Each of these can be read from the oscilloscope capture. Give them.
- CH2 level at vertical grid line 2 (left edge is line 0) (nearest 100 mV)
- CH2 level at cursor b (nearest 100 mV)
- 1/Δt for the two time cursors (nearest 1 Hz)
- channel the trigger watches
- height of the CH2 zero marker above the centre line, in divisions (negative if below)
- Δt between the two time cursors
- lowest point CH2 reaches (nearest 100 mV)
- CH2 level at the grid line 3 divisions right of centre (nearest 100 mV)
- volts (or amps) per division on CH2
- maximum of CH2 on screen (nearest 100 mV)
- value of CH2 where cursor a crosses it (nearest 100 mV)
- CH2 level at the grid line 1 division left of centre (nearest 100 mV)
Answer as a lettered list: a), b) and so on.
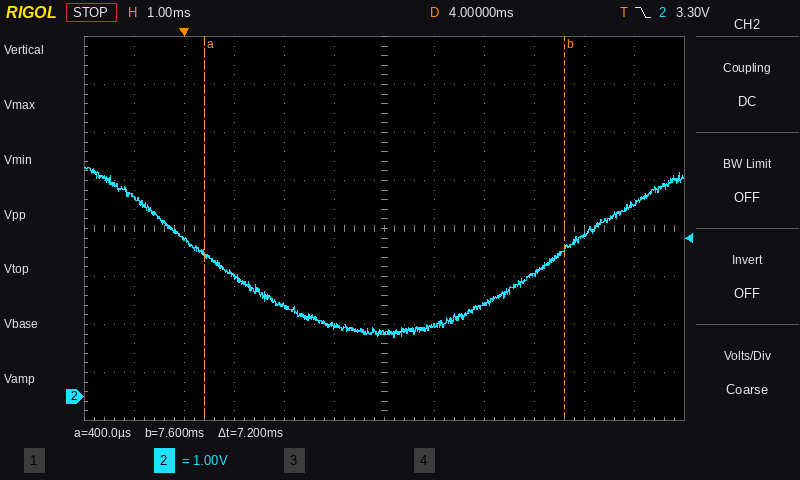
a) 3.3 V
b) 3.1 V
c) 139 Hz
d) CH2
e) -3.5 div
f) 7.2 ms
g) 1.2 V
h) 2.6 V
i) 1 V
j) 4.8 V
k) 3.0 V
l) 1.5 V
